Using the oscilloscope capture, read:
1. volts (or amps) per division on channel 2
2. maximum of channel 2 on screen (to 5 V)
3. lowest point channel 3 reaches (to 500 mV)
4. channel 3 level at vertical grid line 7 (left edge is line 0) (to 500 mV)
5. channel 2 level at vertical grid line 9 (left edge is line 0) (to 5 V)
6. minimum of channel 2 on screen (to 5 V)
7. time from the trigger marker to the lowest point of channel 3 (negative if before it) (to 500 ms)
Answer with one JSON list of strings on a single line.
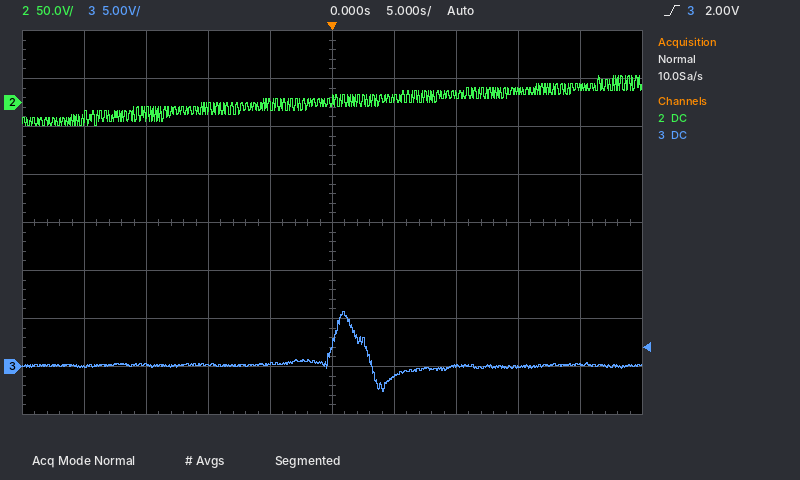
["50 V", "30 V", "-2.5 V", "0.0 V", "15 V", "-25 V", "+4.0 s"]
